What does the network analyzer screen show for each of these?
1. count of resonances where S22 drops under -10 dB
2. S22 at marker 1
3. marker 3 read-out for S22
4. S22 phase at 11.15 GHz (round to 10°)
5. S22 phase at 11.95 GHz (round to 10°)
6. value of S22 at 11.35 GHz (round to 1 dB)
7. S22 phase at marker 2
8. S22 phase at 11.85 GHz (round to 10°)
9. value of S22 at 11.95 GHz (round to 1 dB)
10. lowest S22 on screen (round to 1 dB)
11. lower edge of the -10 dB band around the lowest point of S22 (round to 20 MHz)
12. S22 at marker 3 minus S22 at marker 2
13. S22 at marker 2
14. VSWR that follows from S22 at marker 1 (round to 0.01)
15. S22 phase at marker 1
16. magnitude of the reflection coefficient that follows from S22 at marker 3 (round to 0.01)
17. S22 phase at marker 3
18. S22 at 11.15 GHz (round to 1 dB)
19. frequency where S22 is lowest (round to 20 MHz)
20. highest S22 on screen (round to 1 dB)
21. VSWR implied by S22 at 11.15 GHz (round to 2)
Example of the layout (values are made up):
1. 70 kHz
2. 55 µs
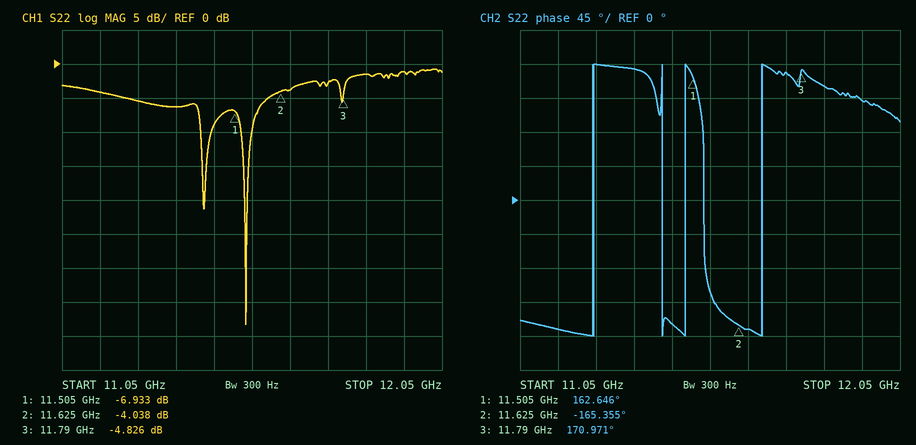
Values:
1. 2
2. -6.933 dB
3. -4.826 dB
4. -170°
5. 130°
6. -6 dB
7. -165.355°
8. 150°
9. -1 dB
10. -38 dB
11. 11.52 GHz
12. -0.788 dB
13. -4.038 dB
14. 2.64
15. 162.646°
16. 0.57
17. 170.971°
18. -4 dB
19. 11.54 GHz
20. -1 dB
21. 4
